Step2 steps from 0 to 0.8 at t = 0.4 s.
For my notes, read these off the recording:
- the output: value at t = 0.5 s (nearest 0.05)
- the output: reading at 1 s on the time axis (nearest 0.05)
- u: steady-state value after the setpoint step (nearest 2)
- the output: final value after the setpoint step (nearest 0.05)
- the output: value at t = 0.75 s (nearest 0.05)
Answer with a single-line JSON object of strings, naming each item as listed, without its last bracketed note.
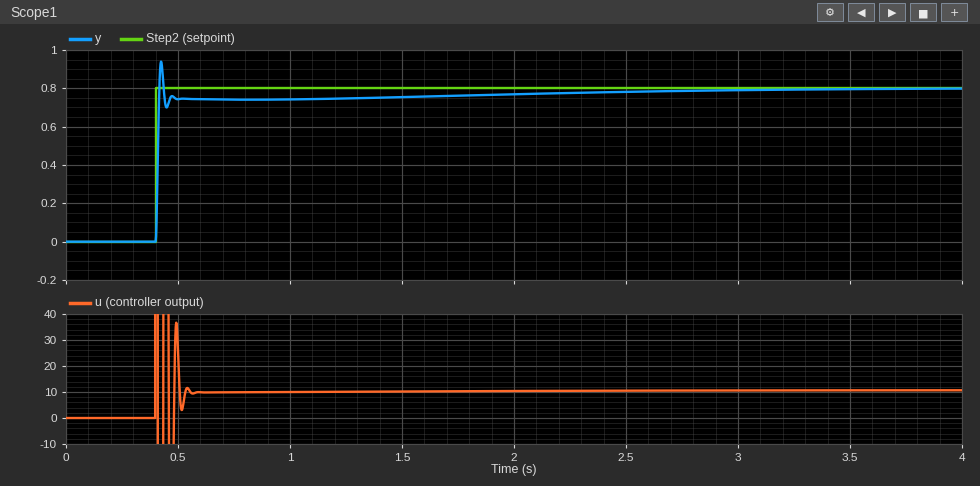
{"the output: value at t = 0.5 s": "0.75", "the output: reading at 1 s on the time axis": "0.75", "u: steady-state value after the setpoint step": "10", "the output: final value after the setpoint step": "0.80", "the output: value at t = 0.75 s": "0.75"}
